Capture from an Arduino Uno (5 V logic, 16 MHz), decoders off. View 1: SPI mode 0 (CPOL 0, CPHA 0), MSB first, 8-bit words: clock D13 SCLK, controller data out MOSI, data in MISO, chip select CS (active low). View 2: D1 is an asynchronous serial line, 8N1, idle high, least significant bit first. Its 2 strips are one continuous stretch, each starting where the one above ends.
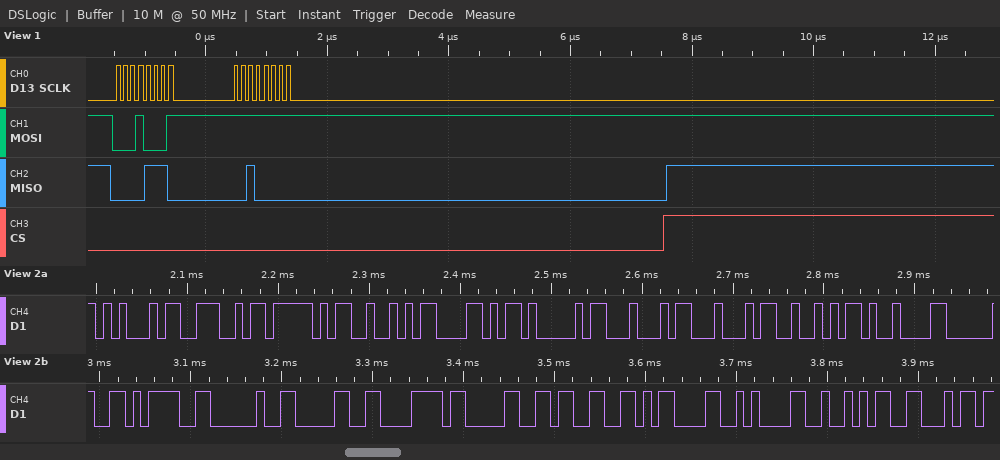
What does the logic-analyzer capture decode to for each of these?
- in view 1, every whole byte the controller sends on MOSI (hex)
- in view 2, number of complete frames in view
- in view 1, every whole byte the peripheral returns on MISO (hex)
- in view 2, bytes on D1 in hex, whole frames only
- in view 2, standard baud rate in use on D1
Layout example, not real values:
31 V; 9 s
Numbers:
0x11 0xFF; 21; 0x0E 0x20; 45 4E 5F 52 58 41 44 44 52 09 20 3D 20 30 78 30 33 0D 0A 52 46; 115200 baud
